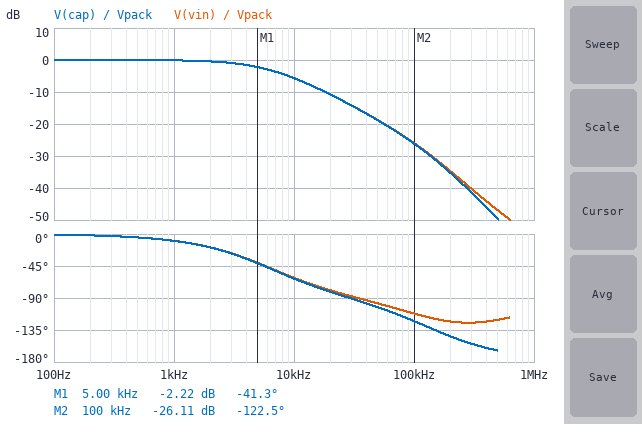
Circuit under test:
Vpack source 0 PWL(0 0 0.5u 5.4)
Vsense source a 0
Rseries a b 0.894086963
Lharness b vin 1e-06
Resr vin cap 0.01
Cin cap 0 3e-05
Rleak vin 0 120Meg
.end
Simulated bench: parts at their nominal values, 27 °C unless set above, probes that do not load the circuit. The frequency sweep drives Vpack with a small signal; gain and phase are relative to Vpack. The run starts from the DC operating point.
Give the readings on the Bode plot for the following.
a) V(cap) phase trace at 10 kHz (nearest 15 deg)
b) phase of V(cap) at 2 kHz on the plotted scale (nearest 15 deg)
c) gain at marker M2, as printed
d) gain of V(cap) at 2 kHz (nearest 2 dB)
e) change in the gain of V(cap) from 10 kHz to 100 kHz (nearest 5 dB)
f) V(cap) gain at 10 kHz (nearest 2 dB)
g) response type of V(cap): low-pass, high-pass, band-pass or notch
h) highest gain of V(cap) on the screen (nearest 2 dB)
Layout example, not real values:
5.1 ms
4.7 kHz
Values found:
-60 deg
-15 deg
-26.11 dB
0 dB
-20 dB
-6 dB
low-pass
0 dB
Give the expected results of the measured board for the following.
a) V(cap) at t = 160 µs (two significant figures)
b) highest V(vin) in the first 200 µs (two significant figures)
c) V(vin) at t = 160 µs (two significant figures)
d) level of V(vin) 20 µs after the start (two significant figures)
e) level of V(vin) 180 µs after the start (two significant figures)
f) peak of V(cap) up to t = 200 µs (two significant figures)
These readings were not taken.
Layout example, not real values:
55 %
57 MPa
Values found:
5.4 V
5.4 V
5.4 V
2.8 V
5.4 V
5.4 V
